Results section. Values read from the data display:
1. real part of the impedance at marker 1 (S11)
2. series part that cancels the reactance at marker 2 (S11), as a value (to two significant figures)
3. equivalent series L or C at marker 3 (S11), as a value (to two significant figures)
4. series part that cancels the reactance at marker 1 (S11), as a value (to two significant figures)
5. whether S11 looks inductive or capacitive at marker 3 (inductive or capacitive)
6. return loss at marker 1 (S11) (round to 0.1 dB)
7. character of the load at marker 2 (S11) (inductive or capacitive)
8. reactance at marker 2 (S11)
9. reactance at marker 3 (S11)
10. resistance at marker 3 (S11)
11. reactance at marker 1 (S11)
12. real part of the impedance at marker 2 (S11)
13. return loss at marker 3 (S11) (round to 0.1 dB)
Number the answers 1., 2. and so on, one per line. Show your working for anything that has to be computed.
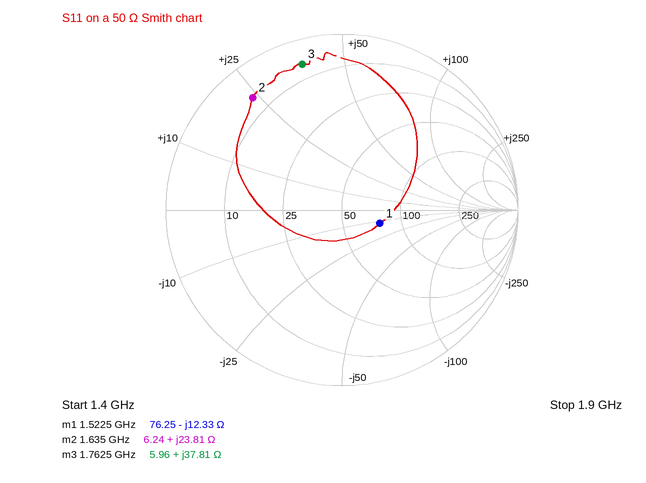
1. 76.25 Ω
2. C = 1/(2π × 1.635 GHz × 23.81 Ω) ≈ 4.1 pF
3. L = 37.81 Ω/(2π × 1.7625 GHz) ≈ 3.4 nH
4. L = 12.33 Ω/(2π × 1.5225 GHz) ≈ 1.3 nH
5. inductive
6. 12.8 dB
7. inductive
8. +23.81 Ω
9. +37.81 Ω
10. 5.96 Ω
11. -12.33 Ω
12. 6.24 Ω
13. 1.3 dB
